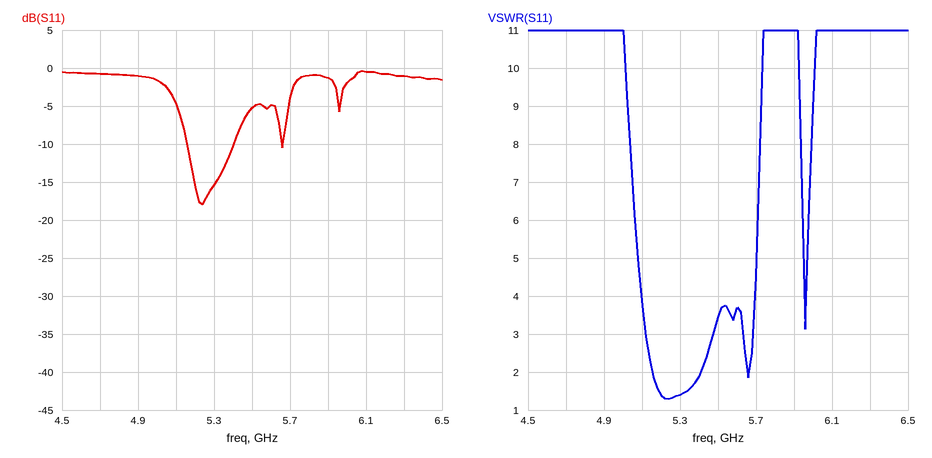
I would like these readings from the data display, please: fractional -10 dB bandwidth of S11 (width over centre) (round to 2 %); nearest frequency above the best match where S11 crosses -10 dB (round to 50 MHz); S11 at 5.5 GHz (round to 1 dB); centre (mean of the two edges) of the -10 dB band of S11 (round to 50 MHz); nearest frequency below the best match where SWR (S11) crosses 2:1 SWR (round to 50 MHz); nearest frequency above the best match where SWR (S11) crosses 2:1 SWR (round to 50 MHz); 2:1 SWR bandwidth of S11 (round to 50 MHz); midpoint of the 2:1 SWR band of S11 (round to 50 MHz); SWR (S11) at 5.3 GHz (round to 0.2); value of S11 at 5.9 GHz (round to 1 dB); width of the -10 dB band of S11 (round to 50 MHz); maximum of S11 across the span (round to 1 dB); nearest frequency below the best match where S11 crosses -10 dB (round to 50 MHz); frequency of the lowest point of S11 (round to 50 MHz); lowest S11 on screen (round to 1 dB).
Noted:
4 %
5.40 GHz
-5 dB
5.30 GHz
5.15 GHz
5.40 GHz
250 MHz
5.30 GHz
1.4
-1 dB
250 MHz
0 dB
5.15 GHz
5.25 GHz
-18 dB
